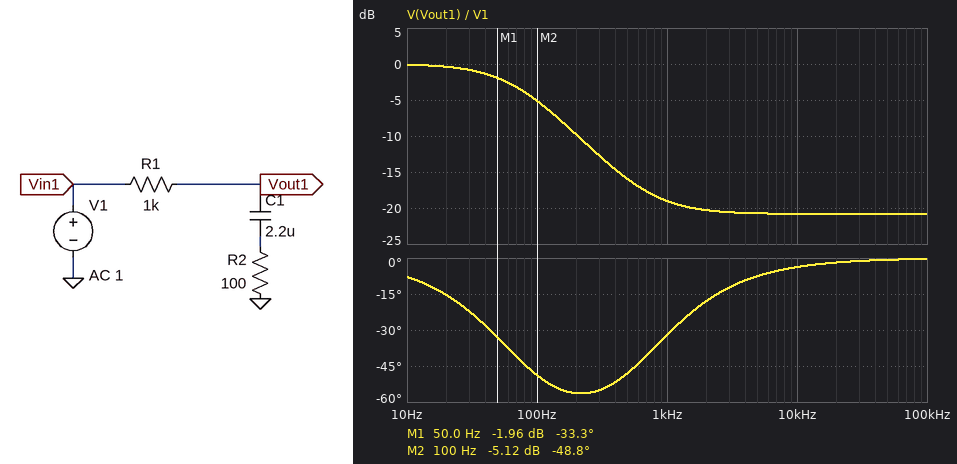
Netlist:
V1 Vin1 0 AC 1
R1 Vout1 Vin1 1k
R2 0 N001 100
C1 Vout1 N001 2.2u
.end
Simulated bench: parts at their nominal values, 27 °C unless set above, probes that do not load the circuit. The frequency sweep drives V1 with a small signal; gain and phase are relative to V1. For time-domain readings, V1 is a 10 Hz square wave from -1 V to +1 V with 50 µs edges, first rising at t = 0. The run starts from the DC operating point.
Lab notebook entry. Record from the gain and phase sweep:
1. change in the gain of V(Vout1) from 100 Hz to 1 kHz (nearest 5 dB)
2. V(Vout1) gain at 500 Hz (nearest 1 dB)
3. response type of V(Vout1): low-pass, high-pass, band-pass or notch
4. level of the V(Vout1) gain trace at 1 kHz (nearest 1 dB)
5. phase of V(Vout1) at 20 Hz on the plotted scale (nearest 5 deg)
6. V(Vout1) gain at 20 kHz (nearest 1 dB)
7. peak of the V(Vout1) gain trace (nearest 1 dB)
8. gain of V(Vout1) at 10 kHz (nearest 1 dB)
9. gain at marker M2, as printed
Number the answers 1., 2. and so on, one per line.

1. -15 dB
2. -16 dB
3. low-pass
4. -19 dB
5. -15 deg
6. -21 dB
7. 0 dB
8. -21 dB
9. -5.12 dB
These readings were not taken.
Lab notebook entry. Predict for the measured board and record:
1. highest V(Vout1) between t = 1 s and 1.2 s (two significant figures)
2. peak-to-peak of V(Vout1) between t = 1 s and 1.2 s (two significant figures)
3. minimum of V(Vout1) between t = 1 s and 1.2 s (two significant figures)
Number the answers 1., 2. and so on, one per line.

1. 1.0 V
2. 2.0 V
3. -1.0 V
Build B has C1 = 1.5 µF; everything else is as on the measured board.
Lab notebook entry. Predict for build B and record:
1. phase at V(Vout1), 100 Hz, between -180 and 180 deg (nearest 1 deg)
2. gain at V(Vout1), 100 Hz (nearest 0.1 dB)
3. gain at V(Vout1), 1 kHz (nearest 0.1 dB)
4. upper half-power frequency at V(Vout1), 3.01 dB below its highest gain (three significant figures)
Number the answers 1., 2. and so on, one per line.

1. -41 deg
2. -3.1 dB
3. -17.6 dB
4. 97.3 Hz
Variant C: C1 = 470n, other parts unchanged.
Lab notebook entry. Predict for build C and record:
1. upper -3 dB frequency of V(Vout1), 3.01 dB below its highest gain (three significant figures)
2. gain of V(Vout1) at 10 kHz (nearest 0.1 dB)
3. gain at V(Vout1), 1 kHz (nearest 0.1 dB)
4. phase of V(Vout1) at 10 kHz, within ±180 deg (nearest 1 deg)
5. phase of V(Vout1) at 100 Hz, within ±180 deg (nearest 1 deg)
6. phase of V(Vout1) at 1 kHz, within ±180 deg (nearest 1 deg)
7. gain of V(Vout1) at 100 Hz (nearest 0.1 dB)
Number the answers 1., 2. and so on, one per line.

1. 310 Hz
2. -20.4 dB
3. -10.3 dB
4. -17 deg
5. -16 deg
6. -56 deg
7. -0.4 dB
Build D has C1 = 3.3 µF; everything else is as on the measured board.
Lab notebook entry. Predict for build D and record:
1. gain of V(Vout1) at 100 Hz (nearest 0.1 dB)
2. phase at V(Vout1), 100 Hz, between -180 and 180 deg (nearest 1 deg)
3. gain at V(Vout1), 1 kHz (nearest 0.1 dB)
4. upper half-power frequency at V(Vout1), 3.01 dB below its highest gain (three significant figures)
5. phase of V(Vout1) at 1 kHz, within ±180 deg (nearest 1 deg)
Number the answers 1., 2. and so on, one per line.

1. -7.7 dB
2. -55 deg
3. -19.9 dB
4. 44.2 Hz
5. -23 deg
